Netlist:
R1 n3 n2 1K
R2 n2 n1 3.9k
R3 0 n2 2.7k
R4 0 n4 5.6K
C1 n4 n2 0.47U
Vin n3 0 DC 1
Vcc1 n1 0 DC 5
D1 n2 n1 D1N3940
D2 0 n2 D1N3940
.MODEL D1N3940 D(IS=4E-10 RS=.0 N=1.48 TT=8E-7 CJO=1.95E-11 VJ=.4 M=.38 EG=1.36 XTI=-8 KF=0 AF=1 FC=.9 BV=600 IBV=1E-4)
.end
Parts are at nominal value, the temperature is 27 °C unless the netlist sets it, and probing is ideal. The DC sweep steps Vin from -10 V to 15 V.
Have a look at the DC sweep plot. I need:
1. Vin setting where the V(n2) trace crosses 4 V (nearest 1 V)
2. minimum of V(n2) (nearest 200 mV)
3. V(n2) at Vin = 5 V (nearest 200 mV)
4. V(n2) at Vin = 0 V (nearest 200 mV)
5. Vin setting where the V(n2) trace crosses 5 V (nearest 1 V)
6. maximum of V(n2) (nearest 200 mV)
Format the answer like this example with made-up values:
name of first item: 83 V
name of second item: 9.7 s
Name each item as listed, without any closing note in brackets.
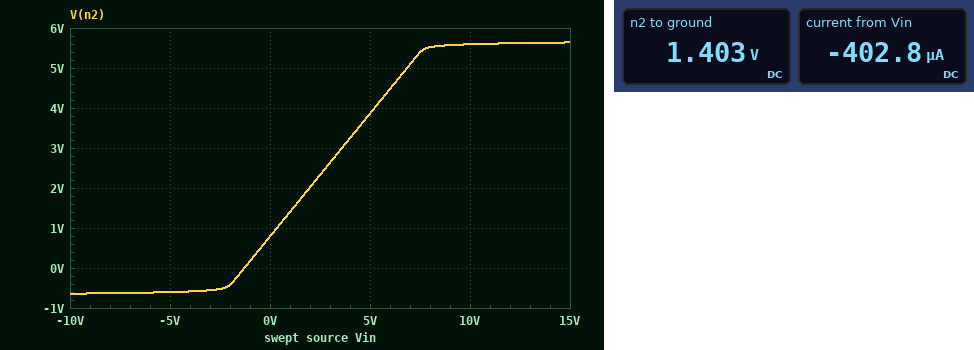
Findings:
Vin setting where the V(n2) trace crosses 4 V: 5 V
minimum of V(n2): -600 mV
V(n2) at Vin = 5 V: 3.8 V
V(n2) at Vin = 0 V: 800 mV
Vin setting where the V(n2) trace crosses 5 V: 7 V
maximum of V(n2): 5.6 V
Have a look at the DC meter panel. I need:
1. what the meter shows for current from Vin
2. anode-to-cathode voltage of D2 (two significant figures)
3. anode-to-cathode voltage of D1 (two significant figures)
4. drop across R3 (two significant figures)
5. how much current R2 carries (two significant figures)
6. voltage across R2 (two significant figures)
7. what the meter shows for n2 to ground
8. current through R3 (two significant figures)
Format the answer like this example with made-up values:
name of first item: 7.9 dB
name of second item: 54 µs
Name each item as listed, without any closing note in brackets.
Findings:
what the meter shows for current from Vin: -402.8 µA
anode-to-cathode voltage of D2: -1.4 V
anode-to-cathode voltage of D1: -3.6 V
drop across R3: 1.4 V
how much current R2 carries: 920 µA
voltage across R2: 3.6 V
what the meter shows for n2 to ground: 1.403 V
current through R3: 520 µA
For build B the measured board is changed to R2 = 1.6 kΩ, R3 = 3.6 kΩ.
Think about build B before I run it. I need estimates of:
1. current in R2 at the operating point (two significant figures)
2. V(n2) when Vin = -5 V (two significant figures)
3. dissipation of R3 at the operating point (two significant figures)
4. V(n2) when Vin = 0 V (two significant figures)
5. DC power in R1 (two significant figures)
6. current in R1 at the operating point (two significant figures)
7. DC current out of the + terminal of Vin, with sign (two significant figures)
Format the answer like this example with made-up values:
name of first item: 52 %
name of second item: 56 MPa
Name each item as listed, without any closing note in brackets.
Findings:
current in R2 at the operating point: 1.8 mA
V(n2) when Vin = -5 V: -560 mV
dissipation of R3 at the operating point: 1.3 mW
V(n2) when Vin = 0 V: 1.6 V
DC power in R1: 1.4 mW
current in R1 at the operating point: 1.2 mA
DC current out of the + terminal of Vin, with sign: -1.2 mA
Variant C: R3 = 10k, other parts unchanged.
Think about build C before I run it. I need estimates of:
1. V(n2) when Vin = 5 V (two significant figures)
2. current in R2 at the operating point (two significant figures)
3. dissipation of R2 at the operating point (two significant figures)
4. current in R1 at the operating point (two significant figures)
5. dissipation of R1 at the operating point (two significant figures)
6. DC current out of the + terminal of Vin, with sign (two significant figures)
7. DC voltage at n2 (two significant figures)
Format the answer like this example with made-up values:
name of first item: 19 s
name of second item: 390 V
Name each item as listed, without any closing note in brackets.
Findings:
V(n2) when Vin = 5 V: 4.6 V
current in R2 at the operating point: 850 µA
dissipation of R2 at the operating point: 2.8 mW
current in R1 at the operating point: 680 µA
dissipation of R1 at the operating point: 470 µW
DC current out of the + terminal of Vin, with sign: -680 µA
DC voltage at n2: 1.7 V
